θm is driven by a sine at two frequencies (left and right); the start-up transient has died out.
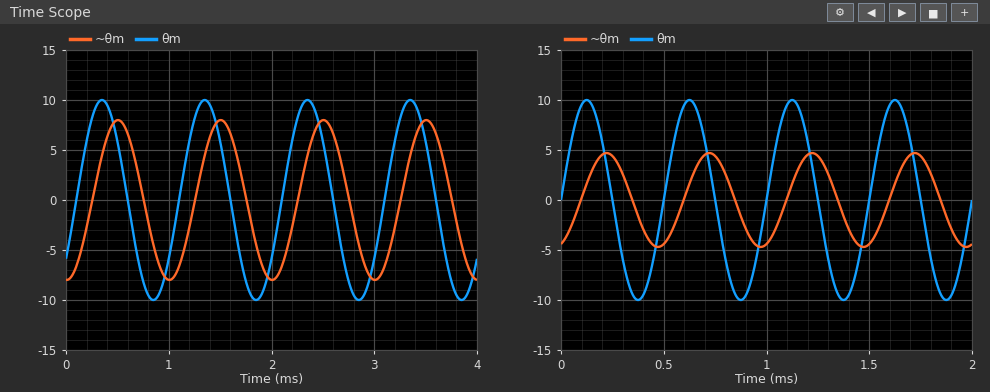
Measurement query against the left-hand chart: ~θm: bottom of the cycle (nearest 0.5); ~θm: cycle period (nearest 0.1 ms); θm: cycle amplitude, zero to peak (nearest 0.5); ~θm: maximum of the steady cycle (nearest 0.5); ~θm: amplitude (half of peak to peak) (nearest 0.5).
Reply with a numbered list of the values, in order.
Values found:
1. -8.0
2. 1.0 ms
3. 10.0
4. 8.0
5. 8.0
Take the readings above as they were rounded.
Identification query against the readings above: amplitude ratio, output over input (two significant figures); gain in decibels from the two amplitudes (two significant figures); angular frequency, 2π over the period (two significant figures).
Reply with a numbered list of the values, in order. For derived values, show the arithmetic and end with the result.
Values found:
1. 8 / 10 = 0.80
2. 20 log10(8 / 10) = -1.9 dB
3. 2π / 1 = 6.3 rad/ms
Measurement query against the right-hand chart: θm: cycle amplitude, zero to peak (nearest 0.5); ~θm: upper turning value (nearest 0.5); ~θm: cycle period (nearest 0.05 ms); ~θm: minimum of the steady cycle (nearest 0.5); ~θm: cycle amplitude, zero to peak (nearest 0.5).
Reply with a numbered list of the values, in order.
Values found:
1. 10.0
2. 4.5
3. 0.50 ms
4. -4.5
5. 4.5
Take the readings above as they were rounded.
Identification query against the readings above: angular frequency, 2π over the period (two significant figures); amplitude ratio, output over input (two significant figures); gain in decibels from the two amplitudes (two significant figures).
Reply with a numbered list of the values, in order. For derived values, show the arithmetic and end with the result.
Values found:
1. 2π / 0.5 = 13 rad/ms
2. 4.5 / 10 = 0.45
3. 20 log10(4.5 / 10) = -6.9 dB
